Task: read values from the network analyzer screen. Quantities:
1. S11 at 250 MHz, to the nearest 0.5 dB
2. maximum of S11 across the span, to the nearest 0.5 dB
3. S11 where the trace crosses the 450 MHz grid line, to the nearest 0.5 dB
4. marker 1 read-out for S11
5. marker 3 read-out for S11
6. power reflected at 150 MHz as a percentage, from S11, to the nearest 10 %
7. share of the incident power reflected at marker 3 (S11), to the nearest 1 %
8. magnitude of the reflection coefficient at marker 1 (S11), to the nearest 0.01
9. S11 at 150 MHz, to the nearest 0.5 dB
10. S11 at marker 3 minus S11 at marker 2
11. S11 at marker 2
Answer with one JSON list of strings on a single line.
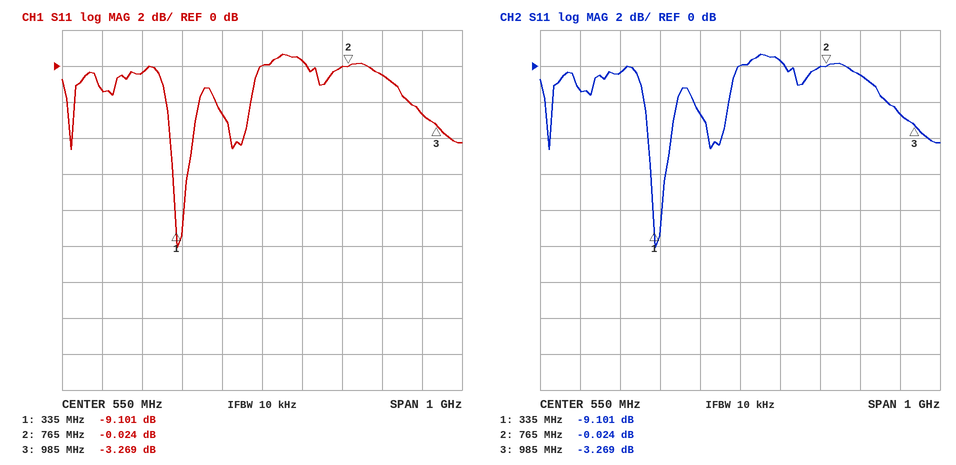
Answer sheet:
["-0.5 dB", "0.5 dB", "-2.5 dB", "-9.101 dB", "-3.269 dB", "70 %", "47 %", "0.35", "-1.5 dB", "-3.245 dB", "-0.024 dB"]
